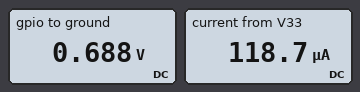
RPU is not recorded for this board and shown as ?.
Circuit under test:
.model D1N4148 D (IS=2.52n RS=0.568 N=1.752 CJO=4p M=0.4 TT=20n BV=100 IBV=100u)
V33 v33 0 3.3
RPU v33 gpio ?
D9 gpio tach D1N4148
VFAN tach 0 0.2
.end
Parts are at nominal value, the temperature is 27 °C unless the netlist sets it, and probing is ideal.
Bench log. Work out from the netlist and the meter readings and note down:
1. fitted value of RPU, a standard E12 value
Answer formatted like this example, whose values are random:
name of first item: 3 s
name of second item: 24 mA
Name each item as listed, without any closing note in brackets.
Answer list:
fitted value of RPU, a standard E12 value: 22 kΩ
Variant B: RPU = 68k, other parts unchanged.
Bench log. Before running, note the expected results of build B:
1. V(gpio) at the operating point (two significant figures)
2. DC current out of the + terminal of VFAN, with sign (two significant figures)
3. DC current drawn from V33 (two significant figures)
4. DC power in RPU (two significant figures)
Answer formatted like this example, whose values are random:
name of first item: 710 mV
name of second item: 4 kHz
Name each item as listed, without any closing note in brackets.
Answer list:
V(gpio) at the operating point: 640 mV
DC current out of the + terminal of VFAN, with sign: -39 µA
DC current drawn from V33: 39 µA
DC power in RPU: 100 µW
